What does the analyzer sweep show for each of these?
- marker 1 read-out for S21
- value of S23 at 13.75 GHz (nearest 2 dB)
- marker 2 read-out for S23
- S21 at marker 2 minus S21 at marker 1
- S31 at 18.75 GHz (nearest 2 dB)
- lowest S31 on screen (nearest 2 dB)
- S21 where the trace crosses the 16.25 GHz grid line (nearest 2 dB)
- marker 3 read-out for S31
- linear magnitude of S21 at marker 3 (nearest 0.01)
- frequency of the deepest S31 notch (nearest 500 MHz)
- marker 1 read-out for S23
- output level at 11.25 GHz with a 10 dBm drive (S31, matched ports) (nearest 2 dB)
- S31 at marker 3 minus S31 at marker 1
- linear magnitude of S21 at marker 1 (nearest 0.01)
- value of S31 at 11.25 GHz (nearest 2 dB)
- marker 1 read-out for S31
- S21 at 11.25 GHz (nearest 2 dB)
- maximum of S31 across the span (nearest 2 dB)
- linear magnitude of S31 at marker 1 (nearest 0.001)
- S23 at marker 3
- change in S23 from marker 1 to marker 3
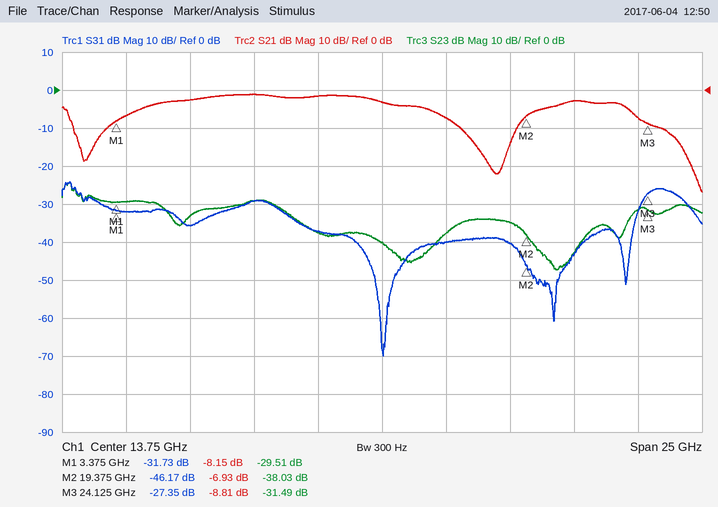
-8.15 dB
-40 dB
-38.03 dB
1.22 dB
-40 dB
-70 dB
-8 dB
-27.35 dB
0.36
14.0 GHz
-29.51 dB
-28 dBm
4.38 dB
0.39
-38 dB
-31.73 dB
-2 dB
-24 dB
0.026
-31.49 dB
-1.98 dB
